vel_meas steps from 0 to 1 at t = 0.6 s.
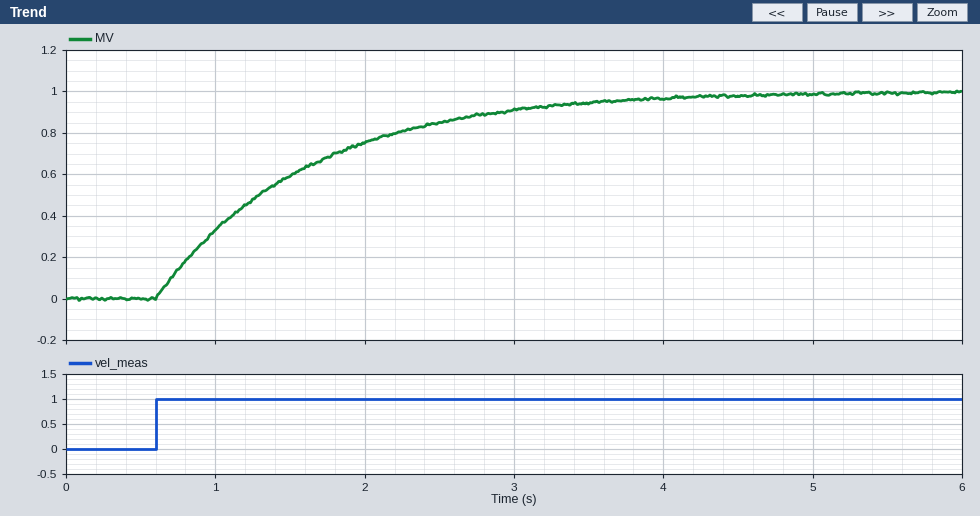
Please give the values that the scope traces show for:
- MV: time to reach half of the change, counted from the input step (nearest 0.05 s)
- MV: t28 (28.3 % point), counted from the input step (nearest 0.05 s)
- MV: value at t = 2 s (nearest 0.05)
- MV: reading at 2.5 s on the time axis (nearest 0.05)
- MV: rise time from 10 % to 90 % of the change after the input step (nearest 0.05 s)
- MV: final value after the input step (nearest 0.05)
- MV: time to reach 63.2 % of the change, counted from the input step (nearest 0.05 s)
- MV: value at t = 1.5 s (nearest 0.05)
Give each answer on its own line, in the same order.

0.70 s
0.35 s
0.75
0.85
2.20 s
1.00
1.00 s
0.60
